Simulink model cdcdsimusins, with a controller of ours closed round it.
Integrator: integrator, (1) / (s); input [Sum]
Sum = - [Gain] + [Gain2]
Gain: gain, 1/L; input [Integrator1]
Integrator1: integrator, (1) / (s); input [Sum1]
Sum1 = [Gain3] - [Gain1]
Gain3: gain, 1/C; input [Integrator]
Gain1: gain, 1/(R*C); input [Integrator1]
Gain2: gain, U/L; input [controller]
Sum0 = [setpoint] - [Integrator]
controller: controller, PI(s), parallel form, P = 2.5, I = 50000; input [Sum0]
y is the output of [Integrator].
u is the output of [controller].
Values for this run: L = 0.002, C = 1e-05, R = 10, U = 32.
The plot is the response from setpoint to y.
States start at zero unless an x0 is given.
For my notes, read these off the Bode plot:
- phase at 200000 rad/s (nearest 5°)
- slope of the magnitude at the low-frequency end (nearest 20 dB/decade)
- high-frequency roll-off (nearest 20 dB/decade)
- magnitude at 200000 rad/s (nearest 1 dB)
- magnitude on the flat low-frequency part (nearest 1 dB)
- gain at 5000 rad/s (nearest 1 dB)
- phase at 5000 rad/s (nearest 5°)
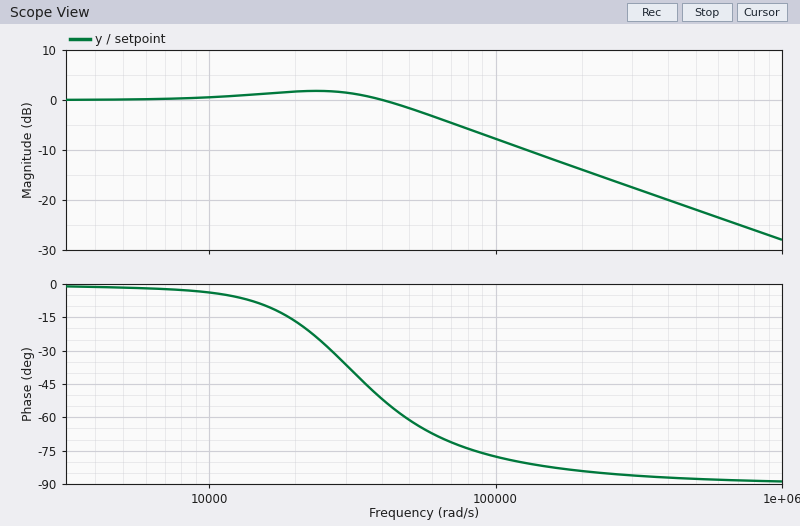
-85°
0 dB/decade
-20 dB/decade
-14 dB
0 dB
0 dB
0°
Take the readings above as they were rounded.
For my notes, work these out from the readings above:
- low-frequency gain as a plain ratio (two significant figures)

1.0
